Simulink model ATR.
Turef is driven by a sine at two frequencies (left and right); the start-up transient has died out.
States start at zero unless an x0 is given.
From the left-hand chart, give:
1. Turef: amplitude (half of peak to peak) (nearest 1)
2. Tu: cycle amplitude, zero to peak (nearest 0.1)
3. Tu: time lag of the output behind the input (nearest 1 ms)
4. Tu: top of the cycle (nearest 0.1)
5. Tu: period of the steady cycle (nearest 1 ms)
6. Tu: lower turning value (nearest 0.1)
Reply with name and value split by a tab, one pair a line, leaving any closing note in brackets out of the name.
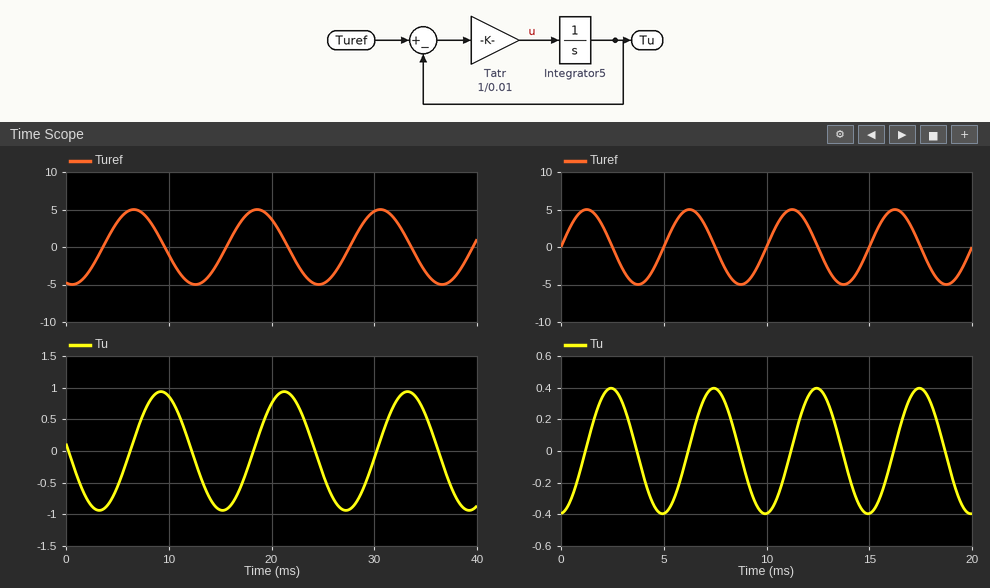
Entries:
Turef: amplitude (half of peak to peak)	5
Tu: cycle amplitude, zero to peak	0.9
Tu: time lag of the output behind the input	3 ms
Tu: top of the cycle	0.9
Tu: period of the steady cycle	12 ms
Tu: lower turning value	-0.9
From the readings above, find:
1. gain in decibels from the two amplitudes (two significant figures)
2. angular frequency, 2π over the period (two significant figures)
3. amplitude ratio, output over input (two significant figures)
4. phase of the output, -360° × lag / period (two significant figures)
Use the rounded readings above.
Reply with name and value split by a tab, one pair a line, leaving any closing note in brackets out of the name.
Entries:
gain in decibels from the two amplitudes	-15 dB
angular frequency, 2π over the period	0.52 rad/ms
amplitude ratio, output over input	0.18
phase of the output, -360° × lag / period	-90°
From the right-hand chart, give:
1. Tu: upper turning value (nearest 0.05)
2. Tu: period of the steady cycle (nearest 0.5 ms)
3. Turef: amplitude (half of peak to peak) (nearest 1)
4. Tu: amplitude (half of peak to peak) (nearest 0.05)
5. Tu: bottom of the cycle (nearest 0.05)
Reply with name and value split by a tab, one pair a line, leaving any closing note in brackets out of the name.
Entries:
Tu: upper turning value	0.40
Tu: period of the steady cycle	5.0 ms
Turef: amplitude (half of peak to peak)	5
Tu: amplitude (half of peak to peak)	0.40
Tu: bottom of the cycle	-0.40
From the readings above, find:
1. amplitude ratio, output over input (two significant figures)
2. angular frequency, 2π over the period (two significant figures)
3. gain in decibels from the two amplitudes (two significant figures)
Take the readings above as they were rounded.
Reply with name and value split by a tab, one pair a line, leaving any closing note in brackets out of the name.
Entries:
amplitude ratio, output over input	0.080
angular frequency, 2π over the period	1.3 rad/ms
gain in decibels from the two amplitudes	-22 dB
